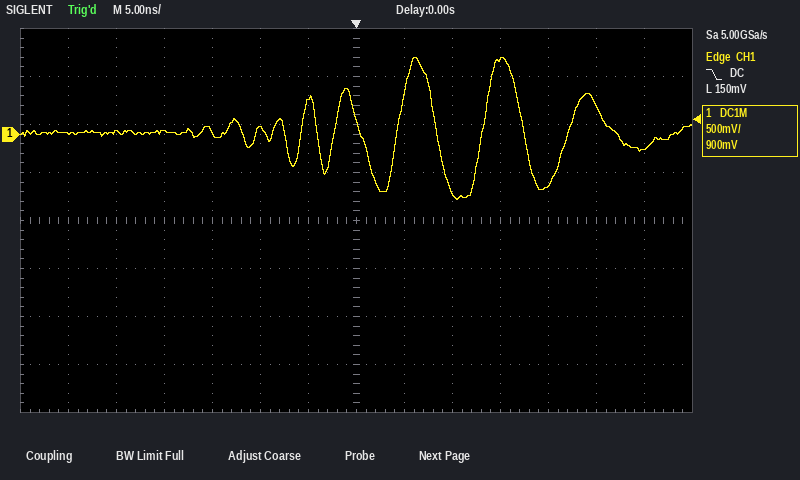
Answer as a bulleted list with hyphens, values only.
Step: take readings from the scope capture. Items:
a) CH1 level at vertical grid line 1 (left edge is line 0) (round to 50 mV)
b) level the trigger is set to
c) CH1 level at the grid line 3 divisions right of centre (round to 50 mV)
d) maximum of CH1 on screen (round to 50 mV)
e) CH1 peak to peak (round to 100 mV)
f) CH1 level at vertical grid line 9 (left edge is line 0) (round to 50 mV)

- 0 mV
- 150 mV
- 800 mV
- 800 mV
- 1.50 V
- -600 mV
